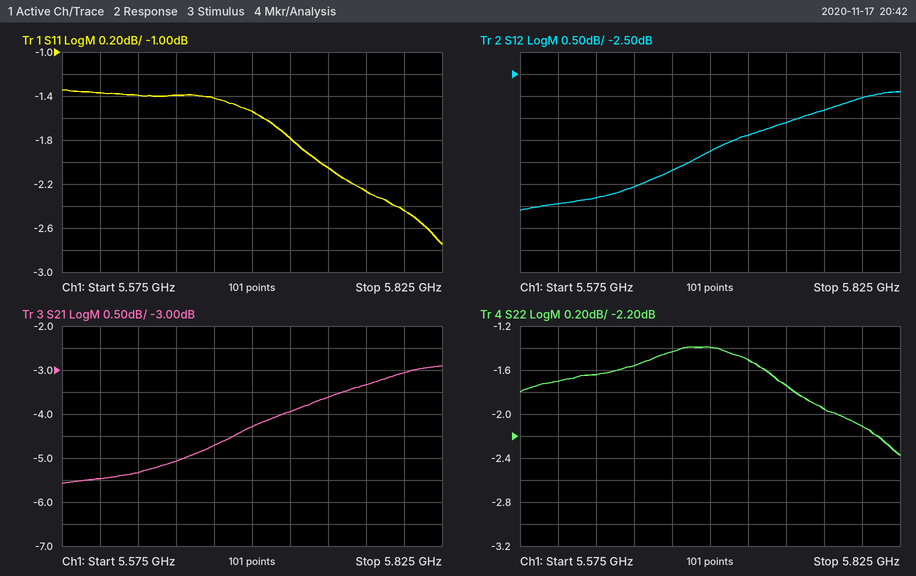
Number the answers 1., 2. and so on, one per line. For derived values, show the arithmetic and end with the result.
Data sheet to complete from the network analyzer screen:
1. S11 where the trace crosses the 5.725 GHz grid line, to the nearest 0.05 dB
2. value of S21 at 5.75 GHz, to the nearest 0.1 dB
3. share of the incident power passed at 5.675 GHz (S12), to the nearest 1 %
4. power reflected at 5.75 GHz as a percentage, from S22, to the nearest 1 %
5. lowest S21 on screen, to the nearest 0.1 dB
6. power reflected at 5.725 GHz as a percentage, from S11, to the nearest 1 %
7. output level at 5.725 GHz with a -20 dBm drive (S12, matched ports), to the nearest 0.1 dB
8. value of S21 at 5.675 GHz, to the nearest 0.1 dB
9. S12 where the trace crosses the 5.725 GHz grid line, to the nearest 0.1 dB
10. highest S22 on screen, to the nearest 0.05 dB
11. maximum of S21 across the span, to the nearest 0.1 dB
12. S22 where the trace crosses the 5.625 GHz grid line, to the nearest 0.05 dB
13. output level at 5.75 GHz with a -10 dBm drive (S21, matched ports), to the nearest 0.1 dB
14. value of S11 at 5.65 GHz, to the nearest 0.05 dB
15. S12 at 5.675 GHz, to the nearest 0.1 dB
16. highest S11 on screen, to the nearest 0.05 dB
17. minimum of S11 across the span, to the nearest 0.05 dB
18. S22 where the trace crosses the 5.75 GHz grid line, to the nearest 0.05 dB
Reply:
1. -1.80 dB
2. -3.6 dB
3. 10^(-4.7/10) ≈ 34 %
4. 10^(-1.75/10) ≈ 67 %
5. -5.6 dB
6. 10^(-1.8/10) ≈ 66 %
7. -20 dBm + (-3.9 dB) = -23.9 dBm
8. -4.7 dB
9. -3.9 dB
10. -1.40 dB
11. -2.9 dB
12. -1.65 dB
13. -10 dBm + (-3.6 dB) = -13.6 dBm
14. -1.40 dB
15. -4.7 dB
16. -1.35 dB
17. -2.75 dB
18. -1.75 dB
